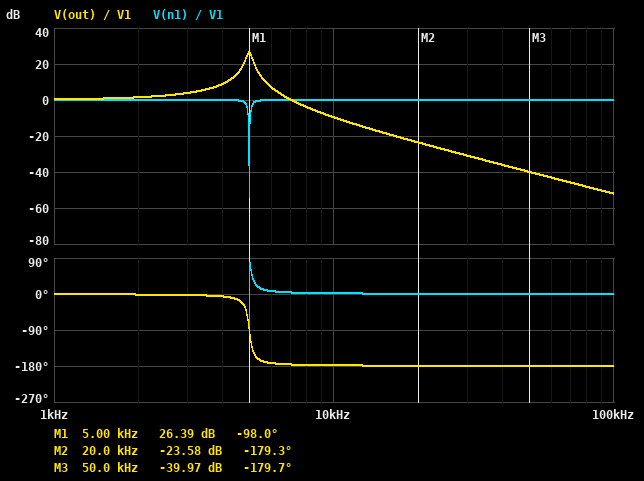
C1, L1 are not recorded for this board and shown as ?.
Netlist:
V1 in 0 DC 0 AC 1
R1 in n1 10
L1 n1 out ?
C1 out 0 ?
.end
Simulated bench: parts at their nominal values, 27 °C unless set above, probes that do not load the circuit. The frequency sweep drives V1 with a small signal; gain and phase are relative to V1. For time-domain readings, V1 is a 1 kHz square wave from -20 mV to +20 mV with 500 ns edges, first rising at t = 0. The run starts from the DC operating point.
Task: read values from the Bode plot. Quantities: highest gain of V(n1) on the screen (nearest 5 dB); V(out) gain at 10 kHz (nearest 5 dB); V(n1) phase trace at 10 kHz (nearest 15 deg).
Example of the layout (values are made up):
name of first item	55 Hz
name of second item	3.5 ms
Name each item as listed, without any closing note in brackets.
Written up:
highest gain of V(n1) on the screen	0 dB
V(out) gain at 10 kHz	-10 dB
V(n1) phase trace at 10 kHz	0 deg
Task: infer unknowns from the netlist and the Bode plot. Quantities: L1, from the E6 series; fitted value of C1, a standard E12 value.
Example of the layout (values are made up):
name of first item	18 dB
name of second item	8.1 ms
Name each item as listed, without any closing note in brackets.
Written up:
L1, from the E6 series	6.8 mH
fitted value of C1, a standard E12 value	150 nF
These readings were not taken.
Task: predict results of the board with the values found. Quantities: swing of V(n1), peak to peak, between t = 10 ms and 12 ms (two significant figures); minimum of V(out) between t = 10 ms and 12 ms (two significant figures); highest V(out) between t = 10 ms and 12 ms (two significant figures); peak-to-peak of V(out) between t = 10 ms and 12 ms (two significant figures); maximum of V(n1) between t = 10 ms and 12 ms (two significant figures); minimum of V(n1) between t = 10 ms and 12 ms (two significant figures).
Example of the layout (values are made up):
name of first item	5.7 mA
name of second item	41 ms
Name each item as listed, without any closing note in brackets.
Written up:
swing of V(n1), peak to peak, between t = 10 ms and 12 ms	51 mV
minimum of V(out) between t = 10 ms and 12 ms	-140 mV
highest V(out) between t = 10 ms and 12 ms	140 mV
peak-to-peak of V(out) between t = 10 ms and 12 ms	280 mV
maximum of V(n1) between t = 10 ms and 12 ms	25 mV
minimum of V(n1) between t = 10 ms and 12 ms	-25 mV
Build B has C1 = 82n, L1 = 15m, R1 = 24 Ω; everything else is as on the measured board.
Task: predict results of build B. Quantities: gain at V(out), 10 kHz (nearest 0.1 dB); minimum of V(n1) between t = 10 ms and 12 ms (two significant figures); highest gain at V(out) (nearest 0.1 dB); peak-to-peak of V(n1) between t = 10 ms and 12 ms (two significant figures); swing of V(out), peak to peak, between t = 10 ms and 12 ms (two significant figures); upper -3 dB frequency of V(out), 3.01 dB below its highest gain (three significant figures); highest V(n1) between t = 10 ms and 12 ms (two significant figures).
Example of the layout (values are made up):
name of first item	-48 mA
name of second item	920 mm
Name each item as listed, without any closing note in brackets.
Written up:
gain at V(out), 10 kHz	-11.7 dB
minimum of V(n1) between t = 10 ms and 12 ms	-22 mV
highest gain at V(out)	25.0 dB
peak-to-peak of V(n1) between t = 10 ms and 12 ms	43 mV
swing of V(out), peak to peak, between t = 10 ms and 12 ms	100 mV
upper -3 dB frequency of V(out), 3.01 dB below its highest gain	4.66 kHz
highest V(n1) between t = 10 ms and 12 ms	22 mV
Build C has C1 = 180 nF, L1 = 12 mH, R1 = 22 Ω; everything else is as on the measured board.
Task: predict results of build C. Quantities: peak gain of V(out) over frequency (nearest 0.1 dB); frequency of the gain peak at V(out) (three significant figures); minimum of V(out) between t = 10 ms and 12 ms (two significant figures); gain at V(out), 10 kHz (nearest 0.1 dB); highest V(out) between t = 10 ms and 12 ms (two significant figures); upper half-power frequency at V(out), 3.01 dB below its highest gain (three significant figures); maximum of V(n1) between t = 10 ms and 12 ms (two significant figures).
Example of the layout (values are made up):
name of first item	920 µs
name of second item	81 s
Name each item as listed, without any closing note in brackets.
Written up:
peak gain of V(out) over frequency	21.4 dB
frequency of the gain peak at V(out)	3.42 kHz
minimum of V(out) between t = 10 ms and 12 ms	-54 mV
gain at V(out), 10 kHz	-17.5 dB
highest V(out) between t = 10 ms and 12 ms	54 mV
upper half-power frequency at V(out), 3.01 dB below its highest gain	3.56 kHz
maximum of V(n1) between t = 10 ms and 12 ms	23 mV
